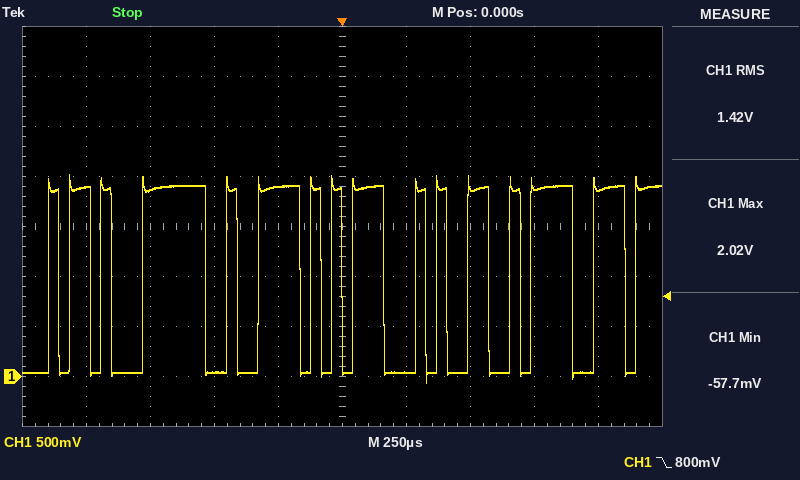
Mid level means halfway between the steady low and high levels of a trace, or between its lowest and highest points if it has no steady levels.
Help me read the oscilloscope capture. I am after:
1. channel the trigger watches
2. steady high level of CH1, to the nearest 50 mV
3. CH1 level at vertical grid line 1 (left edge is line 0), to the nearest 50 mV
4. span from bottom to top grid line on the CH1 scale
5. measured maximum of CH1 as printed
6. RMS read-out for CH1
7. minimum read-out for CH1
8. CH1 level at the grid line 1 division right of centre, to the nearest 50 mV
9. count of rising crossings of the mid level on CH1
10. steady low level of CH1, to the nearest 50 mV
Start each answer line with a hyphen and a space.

- CH1
- 1.90 V
- 1.90 V
- 4 V
- 2.02 V
- 1.42 V
- -57.7 mV
- 50 mV
- 16
- 50 mV
